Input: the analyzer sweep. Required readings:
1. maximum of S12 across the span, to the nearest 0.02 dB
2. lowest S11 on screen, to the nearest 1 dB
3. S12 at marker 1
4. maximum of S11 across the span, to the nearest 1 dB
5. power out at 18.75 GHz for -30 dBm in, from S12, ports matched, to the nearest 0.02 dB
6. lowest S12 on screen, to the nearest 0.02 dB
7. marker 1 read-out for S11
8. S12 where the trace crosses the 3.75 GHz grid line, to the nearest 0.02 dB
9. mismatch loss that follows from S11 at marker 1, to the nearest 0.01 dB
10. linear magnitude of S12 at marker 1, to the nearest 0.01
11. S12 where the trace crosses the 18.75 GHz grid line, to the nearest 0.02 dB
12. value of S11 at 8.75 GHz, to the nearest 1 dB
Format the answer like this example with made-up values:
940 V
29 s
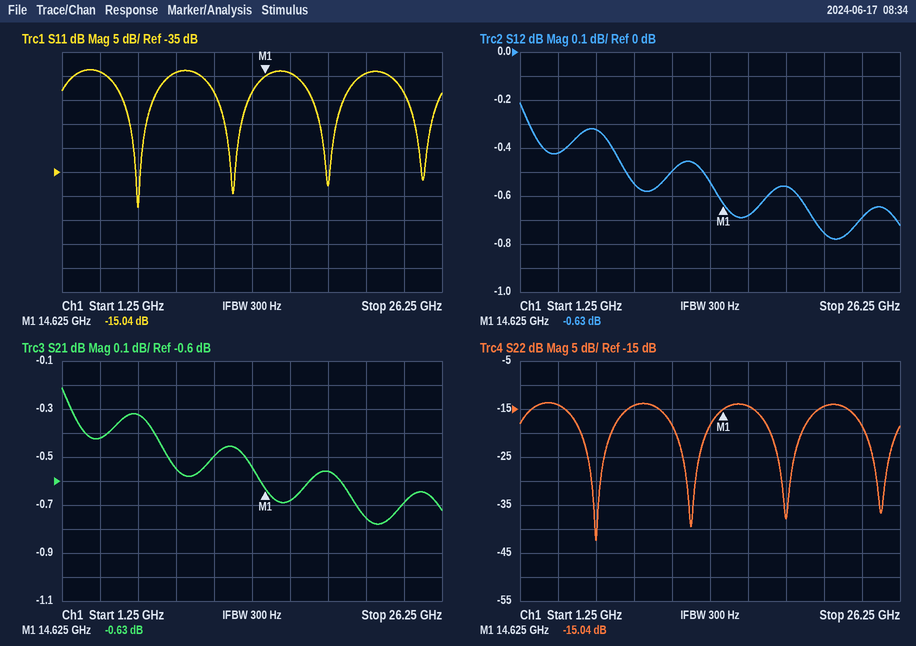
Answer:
-0.22 dB
-42 dB
-0.63 dB
-14 dB
-30.56 dBm
-0.78 dB
-15.04 dB
-0.42 dB
0.14 dB
0.93
-0.56 dB
-14 dB
